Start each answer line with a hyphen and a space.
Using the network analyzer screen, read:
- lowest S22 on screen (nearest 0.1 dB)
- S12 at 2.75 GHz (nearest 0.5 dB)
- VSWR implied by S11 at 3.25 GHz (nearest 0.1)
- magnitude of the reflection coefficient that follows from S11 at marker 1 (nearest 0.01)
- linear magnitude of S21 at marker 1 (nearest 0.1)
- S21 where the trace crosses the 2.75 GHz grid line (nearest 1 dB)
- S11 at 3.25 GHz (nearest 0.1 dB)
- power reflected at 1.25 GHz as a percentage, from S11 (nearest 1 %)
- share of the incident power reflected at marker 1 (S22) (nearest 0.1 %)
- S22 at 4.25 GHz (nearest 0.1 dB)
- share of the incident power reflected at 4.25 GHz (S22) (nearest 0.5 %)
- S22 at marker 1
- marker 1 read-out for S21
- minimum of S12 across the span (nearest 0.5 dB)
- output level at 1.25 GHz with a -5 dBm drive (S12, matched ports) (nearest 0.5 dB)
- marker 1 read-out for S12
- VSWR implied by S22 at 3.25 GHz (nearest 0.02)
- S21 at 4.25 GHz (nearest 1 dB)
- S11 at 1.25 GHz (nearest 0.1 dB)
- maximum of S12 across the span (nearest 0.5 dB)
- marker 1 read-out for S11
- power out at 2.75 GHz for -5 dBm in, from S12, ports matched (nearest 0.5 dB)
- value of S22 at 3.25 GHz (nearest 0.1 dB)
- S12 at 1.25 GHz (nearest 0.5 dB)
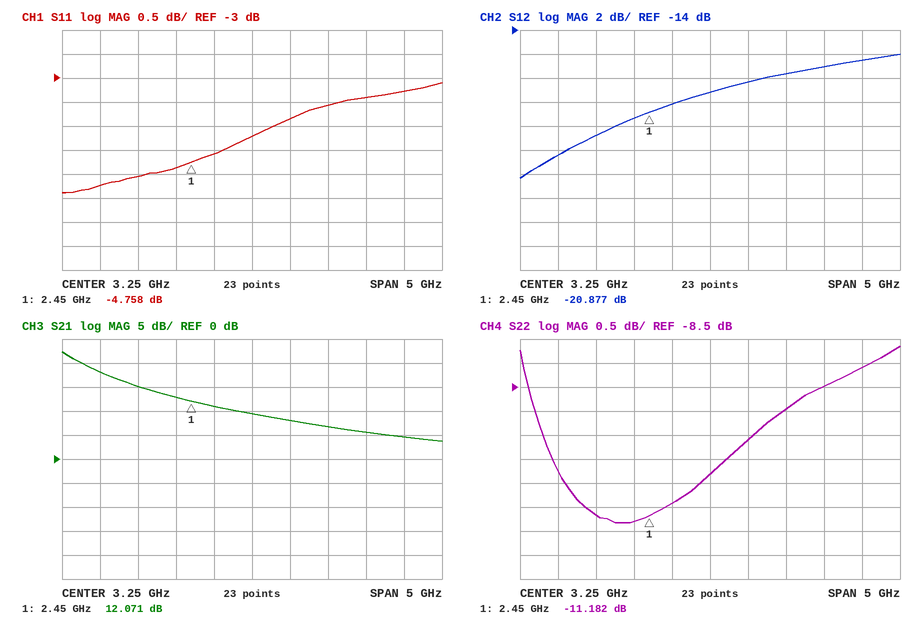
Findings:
- -11.3 dB
- -20.0 dB
- 4.2
- 0.58
- 4.0
- 11 dB
- -4.2 dB
- 30 %
- 7.6 %
- -9.0 dB
- 12.5 %
- -11.182 dB
- 12.071 dB
- -26.5 dB
- -29.5 dBm
- -20.877 dB
- 1.88
- 7 dB
- -5.2 dB
- -16.0 dB
- -4.758 dB
- -25.0 dBm
- -10.3 dB
- -24.5 dB
